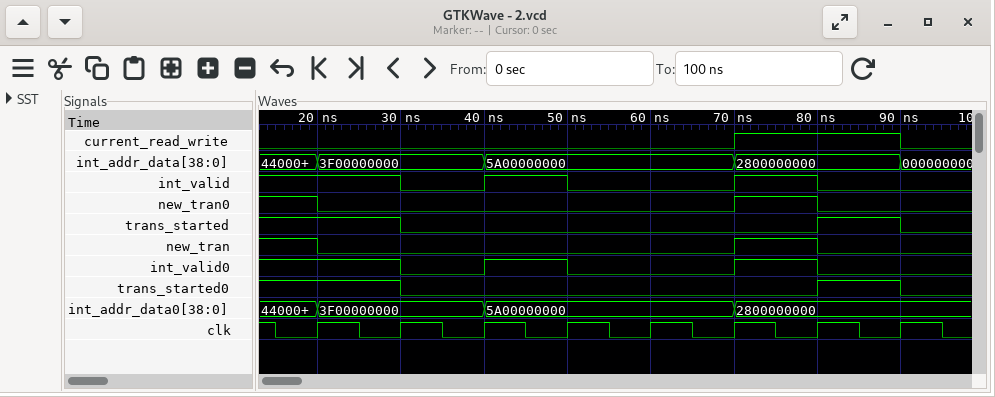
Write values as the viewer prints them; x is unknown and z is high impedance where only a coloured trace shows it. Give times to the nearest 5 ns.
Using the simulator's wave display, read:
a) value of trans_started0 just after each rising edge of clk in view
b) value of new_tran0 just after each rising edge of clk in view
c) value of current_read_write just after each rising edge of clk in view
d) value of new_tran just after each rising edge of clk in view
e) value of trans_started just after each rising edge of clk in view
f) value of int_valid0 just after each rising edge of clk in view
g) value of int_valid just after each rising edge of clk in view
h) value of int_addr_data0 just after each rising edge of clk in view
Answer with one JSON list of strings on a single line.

["1 0 0 0 0 0 1 0", "0 0 0 0 0 1 0 0", "0 0 0 0 0 1 1 0", "0 0 0 0 0 1 0 0", "1 0 0 0 0 0 1 0", "1 0 1 0 0 1 0 0", "1 0 1 0 0 1 0 0", "3F00000000, 3F00000000, 5A00000000, 5A00000000, 5A00000000, 2800000000, 2800000000, 2800000000"]
